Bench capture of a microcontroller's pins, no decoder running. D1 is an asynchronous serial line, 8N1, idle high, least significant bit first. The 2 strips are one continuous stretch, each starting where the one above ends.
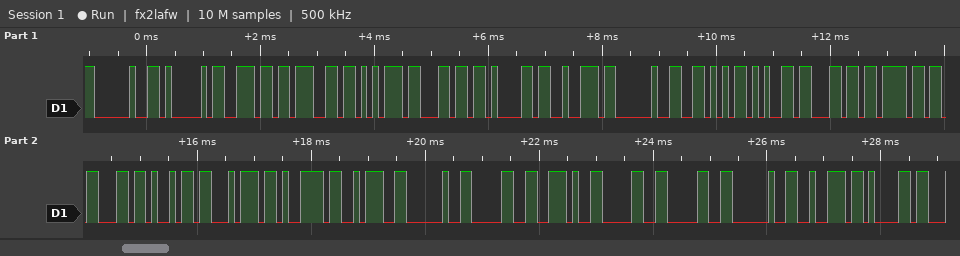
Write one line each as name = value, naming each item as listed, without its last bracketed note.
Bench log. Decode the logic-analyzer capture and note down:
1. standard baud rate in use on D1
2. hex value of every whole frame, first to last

standard baud rate in use on D1 = 9600 baud
hex value of every whole frame, first to last = 0x20 0x41 0x6E 0x67 0x75 0x6C 0x61 0x72 0x20 0x56 0x65 0x6C 0x6F 0x63 0x69 0x74 0x79 0x3A 0x20 0x30 0x2E 0x30 0x30 0x20 0x72 0x61
